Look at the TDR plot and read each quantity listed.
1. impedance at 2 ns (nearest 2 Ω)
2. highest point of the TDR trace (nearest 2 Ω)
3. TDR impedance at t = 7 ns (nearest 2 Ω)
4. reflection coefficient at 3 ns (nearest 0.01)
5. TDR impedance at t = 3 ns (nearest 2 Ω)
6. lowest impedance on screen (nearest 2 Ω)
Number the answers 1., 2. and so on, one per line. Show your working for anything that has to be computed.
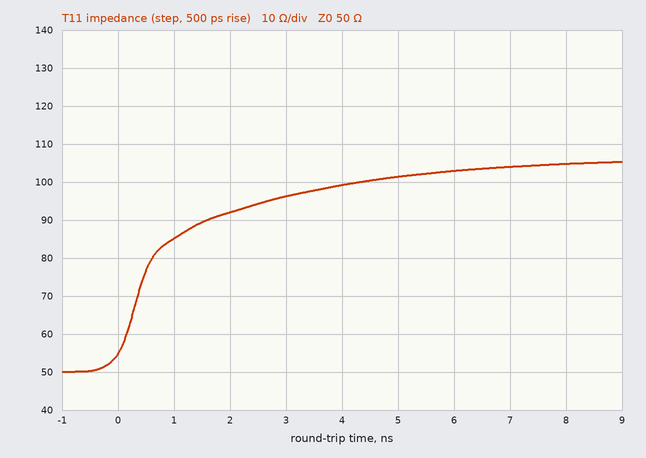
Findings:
1. 92 Ω
2. 106 Ω
3. 104 Ω
4. (96 − 50)/(96 + 50) ≈ +0.32
5. 96 Ω
6. 50 Ω
